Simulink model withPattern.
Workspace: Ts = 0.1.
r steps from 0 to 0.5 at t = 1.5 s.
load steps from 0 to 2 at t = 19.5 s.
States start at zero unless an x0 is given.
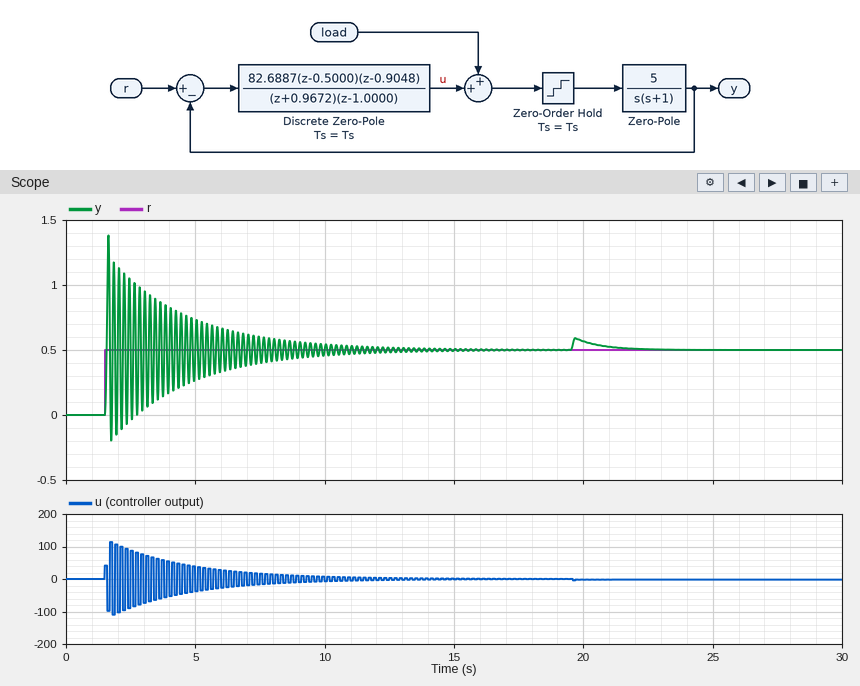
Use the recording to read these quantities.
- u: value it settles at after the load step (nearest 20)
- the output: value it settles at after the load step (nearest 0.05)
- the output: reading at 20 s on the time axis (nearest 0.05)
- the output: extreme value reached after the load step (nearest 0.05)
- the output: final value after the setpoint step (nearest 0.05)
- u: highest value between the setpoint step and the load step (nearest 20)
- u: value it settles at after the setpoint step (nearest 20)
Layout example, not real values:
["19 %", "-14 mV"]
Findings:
["0", "0.50", "0.55", "0.60", "0.50", "120", "0"]
